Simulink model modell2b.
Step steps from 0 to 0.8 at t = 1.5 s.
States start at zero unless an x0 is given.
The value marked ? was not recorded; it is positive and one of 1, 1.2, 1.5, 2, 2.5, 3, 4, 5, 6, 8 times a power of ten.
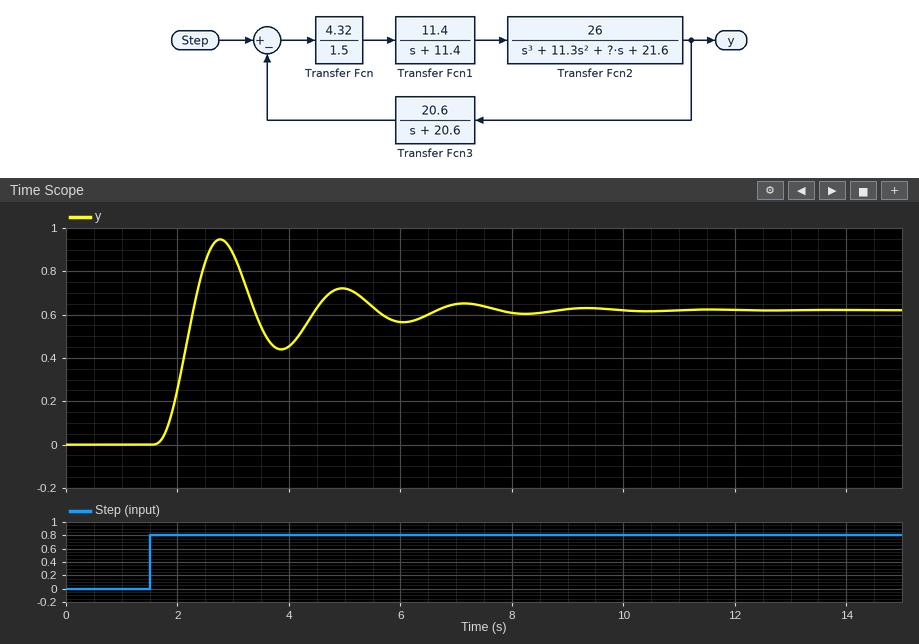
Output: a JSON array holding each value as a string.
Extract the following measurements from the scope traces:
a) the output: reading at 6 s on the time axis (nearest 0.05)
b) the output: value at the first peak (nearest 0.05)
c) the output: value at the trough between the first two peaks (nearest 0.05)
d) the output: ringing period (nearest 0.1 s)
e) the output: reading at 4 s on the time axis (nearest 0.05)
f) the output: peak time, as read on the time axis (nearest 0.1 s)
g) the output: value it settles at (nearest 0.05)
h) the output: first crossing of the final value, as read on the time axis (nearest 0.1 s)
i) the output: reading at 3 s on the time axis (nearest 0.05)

["0.55", "0.95", "0.45", "2.2 s", "0.45", "2.8 s", "0.60", "2.3 s", "0.90"]
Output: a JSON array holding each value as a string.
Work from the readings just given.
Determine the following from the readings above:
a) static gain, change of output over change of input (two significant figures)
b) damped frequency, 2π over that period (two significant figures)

["0.75", "2.9 rad/s"]
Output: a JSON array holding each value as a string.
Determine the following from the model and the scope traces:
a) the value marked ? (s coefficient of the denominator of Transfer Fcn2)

["30"]
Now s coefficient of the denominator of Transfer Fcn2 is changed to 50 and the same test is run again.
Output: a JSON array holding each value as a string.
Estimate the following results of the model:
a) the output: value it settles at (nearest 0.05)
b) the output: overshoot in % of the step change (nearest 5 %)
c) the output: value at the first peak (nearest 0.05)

["0.60", "15 %", "0.70"]
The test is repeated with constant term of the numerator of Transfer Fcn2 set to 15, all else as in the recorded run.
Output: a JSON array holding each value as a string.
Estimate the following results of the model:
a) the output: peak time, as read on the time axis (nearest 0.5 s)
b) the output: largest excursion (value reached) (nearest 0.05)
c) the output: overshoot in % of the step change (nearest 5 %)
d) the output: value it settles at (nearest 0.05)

["3.0 s", "0.70", "30 %", "0.55"]
